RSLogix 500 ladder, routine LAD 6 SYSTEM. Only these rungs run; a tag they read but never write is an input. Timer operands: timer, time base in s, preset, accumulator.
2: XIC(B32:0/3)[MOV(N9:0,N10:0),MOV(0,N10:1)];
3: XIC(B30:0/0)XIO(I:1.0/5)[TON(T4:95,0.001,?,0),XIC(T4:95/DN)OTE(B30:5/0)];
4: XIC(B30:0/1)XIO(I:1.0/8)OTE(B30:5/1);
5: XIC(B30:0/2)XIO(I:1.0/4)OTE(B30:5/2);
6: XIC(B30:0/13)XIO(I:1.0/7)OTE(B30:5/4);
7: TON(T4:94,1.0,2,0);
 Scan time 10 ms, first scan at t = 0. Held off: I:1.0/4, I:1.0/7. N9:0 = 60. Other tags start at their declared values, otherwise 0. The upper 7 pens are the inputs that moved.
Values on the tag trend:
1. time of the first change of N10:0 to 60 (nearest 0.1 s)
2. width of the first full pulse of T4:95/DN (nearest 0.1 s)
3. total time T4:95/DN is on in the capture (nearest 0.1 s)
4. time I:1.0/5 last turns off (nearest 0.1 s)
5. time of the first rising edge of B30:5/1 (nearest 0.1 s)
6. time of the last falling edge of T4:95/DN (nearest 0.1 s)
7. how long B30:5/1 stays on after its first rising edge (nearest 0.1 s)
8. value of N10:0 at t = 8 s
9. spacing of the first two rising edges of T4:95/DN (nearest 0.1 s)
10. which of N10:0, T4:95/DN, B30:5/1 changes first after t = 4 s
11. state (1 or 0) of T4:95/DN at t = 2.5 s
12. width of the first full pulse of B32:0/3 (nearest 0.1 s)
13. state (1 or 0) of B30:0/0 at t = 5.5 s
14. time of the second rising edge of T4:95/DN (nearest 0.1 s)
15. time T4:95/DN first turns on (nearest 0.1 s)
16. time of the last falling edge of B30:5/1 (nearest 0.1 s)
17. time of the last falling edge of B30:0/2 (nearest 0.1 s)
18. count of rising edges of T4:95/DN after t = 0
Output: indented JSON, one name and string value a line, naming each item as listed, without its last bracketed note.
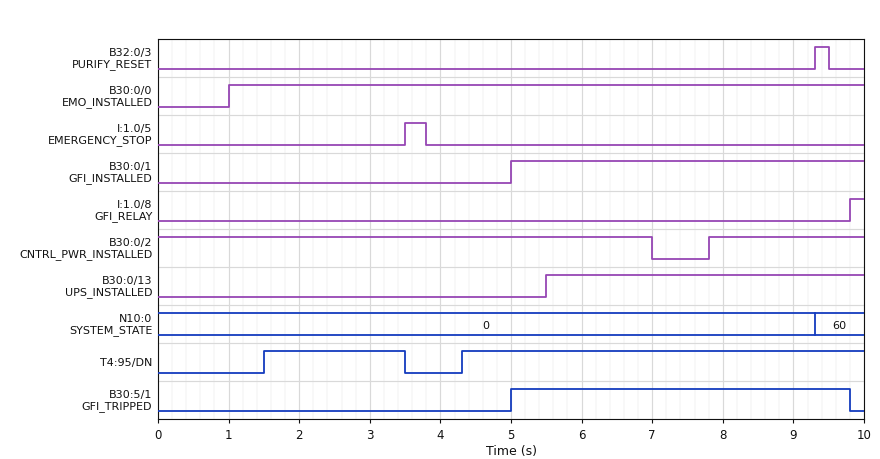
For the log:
{
  "time of the first change of N10:0 to 60": "9.3 s",
  "width of the first full pulse of T4:95/DN": "2.0 s",
  "total time T4:95/DN is on in the capture": "7.7 s",
  "time I:1.0/5 last turns off": "3.8 s",
  "time of the first rising edge of B30:5/1": "5.0 s",
  "time of the last falling edge of T4:95/DN": "3.5 s",
  "how long B30:5/1 stays on after its first rising edge": "4.8 s",
  "value of N10:0 at t = 8 s": "0",
  "spacing of the first two rising edges of T4:95/DN": "2.8 s",
  "which of N10:0, T4:95/DN, B30:5/1 changes first after t = 4 s": "T4:95/DN",
  "state (1 or 0) of T4:95/DN at t = 2.5 s": "1",
  "width of the first full pulse of B32:0/3": "0.2 s",
  "state (1 or 0) of B30:0/0 at t = 5.5 s": "1",
  "time of the second rising edge of T4:95/DN": "4.3 s",
  "time T4:95/DN first turns on": "1.5 s",
  "time of the last falling edge of B30:5/1": "9.8 s",
  "time of the last falling edge of B30:0/2": "7.0 s",
  "count of rising edges of T4:95/DN after t = 0": "2"
}
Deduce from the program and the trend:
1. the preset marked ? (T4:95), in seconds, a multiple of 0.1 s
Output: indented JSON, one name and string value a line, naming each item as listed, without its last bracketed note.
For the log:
{
  "the preset marked ? (T4:95), in seconds, a multiple of 0.1 s": "0.5 s"
}
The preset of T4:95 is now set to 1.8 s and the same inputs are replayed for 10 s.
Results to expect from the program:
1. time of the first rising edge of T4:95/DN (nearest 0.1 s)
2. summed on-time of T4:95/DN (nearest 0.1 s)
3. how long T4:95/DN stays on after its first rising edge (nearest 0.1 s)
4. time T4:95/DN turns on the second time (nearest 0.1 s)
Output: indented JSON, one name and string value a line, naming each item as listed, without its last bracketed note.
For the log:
{
  "time of the first rising edge of T4:95/DN": "2.8 s",
  "summed on-time of T4:95/DN": "5.1 s",
  "how long T4:95/DN stays on after its first rising edge": "0.7 s",
  "time T4:95/DN turns on the second time": "5.6 s"
}
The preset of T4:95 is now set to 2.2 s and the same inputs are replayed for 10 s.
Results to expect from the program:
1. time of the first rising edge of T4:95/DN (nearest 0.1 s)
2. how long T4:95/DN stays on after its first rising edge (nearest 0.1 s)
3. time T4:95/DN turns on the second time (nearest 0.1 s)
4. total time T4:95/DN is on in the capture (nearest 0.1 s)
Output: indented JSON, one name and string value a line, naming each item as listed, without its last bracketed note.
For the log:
{
  "time of the first rising edge of T4:95/DN": "3.2 s",
  "how long T4:95/DN stays on after its first rising edge": "0.3 s",
  "time T4:95/DN turns on the second time": "6.0 s",
  "total time T4:95/DN is on in the capture": "4.3 s"
}
